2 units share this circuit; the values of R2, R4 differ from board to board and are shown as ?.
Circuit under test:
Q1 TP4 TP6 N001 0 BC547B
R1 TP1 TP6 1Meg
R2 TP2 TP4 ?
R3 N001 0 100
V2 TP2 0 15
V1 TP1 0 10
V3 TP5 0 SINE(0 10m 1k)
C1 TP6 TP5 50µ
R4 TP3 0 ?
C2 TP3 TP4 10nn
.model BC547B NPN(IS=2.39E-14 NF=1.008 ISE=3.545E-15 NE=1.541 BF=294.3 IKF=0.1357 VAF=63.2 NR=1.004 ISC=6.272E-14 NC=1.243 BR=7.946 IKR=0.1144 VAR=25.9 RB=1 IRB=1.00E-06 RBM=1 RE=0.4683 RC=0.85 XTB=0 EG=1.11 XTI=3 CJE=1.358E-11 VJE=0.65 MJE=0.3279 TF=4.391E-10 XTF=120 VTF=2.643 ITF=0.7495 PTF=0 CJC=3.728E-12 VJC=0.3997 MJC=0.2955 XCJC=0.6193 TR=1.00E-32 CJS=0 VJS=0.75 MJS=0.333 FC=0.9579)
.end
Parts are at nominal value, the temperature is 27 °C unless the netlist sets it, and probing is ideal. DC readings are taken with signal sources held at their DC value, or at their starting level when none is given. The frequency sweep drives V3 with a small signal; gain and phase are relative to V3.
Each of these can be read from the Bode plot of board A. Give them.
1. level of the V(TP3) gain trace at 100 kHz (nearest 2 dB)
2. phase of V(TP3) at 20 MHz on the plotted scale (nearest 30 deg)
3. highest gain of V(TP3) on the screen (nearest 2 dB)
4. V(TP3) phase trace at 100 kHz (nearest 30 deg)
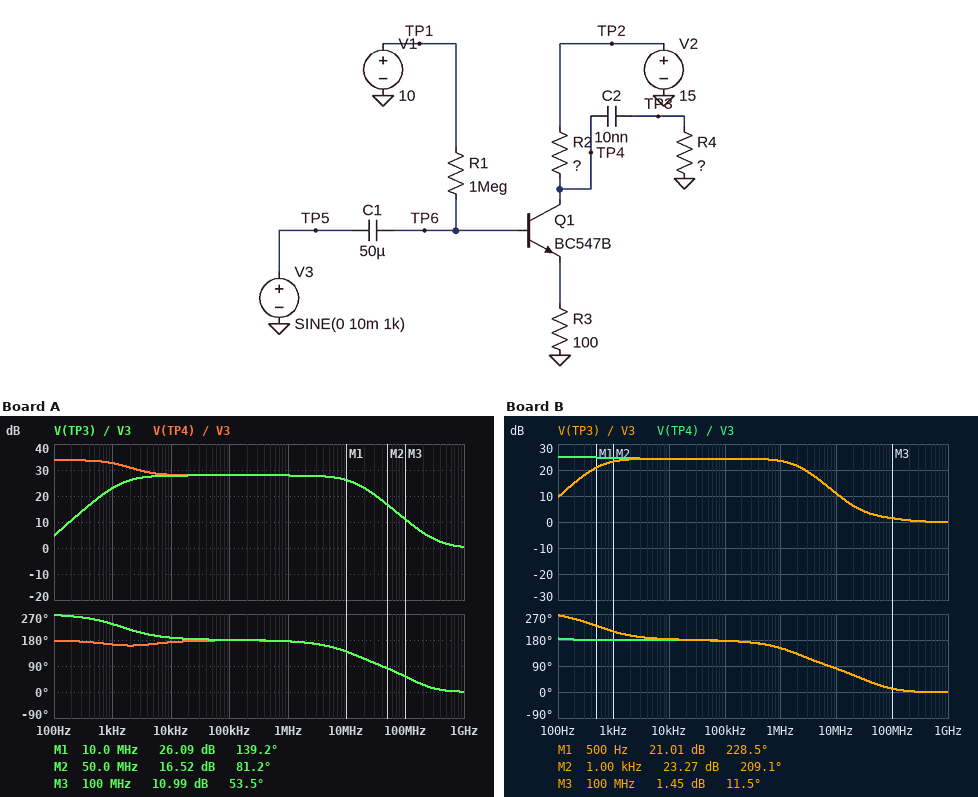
28 dB
120 deg
28 dB
180 deg
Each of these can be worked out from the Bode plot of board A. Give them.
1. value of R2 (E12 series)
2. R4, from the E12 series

5.6 kΩ
5.6 kΩ
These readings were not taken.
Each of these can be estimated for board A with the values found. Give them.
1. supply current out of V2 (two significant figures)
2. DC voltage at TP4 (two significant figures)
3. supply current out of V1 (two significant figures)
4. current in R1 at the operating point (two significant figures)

2.5 mA
810 mV
9.1 µA
9.1 µA
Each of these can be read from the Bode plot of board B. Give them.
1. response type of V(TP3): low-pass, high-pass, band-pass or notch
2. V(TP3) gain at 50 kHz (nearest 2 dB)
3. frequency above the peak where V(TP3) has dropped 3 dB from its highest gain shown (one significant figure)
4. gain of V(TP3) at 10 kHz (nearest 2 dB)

band-pass
24 dB
2 MHz
24 dB
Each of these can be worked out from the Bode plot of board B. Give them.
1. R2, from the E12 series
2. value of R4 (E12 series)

12 kΩ
27 kΩ
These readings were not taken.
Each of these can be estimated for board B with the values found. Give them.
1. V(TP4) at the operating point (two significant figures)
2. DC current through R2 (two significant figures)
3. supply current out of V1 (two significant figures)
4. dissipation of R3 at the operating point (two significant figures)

230 mV
1.2 mA
9.2 µA
150 µW
